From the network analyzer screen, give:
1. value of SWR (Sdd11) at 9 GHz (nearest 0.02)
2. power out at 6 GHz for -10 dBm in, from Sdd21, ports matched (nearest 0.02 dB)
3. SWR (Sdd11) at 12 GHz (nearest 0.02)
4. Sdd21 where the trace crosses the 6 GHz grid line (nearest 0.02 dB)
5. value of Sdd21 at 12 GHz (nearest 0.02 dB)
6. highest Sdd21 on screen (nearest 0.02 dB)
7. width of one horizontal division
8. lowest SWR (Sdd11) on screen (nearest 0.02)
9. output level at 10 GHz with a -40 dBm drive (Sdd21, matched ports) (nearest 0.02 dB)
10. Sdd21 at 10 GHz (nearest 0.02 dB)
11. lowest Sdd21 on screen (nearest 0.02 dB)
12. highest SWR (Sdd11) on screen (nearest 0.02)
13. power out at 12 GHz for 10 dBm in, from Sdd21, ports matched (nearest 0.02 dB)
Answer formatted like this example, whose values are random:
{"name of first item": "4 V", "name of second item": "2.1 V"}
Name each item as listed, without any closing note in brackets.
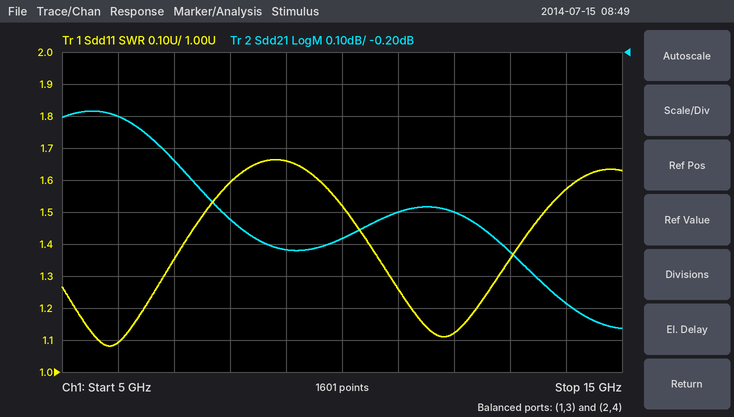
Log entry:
{"value of SWR (Sdd11) at 9 GHz": "1.66", "power out at 6 GHz for -10 dBm in, from Sdd21, ports matched": "-10.40 dBm", "SWR (Sdd11) at 12 GHz": "1.12", "Sdd21 where the trace crosses the 6 GHz grid line": "-0.40 dB", "value of Sdd21 at 12 GHz": "-0.70 dB", "highest Sdd21 on screen": "-0.38 dB", "width of one horizontal division": "1 GHz", "lowest SWR (Sdd11) on screen": "1.08", "output level at 10 GHz with a -40 dBm drive (Sdd21, matched ports)": "-40.78 dBm", "Sdd21 at 10 GHz": "-0.78 dB", "lowest Sdd21 on screen": "-1.06 dB", "highest SWR (Sdd11) on screen": "1.66", "power out at 12 GHz for 10 dBm in, from Sdd21, ports matched": "9.30 dBm"}
